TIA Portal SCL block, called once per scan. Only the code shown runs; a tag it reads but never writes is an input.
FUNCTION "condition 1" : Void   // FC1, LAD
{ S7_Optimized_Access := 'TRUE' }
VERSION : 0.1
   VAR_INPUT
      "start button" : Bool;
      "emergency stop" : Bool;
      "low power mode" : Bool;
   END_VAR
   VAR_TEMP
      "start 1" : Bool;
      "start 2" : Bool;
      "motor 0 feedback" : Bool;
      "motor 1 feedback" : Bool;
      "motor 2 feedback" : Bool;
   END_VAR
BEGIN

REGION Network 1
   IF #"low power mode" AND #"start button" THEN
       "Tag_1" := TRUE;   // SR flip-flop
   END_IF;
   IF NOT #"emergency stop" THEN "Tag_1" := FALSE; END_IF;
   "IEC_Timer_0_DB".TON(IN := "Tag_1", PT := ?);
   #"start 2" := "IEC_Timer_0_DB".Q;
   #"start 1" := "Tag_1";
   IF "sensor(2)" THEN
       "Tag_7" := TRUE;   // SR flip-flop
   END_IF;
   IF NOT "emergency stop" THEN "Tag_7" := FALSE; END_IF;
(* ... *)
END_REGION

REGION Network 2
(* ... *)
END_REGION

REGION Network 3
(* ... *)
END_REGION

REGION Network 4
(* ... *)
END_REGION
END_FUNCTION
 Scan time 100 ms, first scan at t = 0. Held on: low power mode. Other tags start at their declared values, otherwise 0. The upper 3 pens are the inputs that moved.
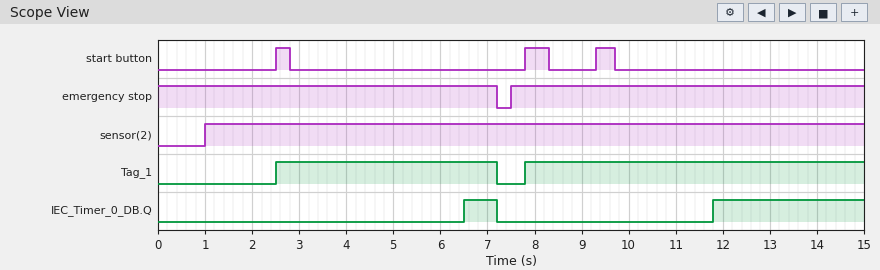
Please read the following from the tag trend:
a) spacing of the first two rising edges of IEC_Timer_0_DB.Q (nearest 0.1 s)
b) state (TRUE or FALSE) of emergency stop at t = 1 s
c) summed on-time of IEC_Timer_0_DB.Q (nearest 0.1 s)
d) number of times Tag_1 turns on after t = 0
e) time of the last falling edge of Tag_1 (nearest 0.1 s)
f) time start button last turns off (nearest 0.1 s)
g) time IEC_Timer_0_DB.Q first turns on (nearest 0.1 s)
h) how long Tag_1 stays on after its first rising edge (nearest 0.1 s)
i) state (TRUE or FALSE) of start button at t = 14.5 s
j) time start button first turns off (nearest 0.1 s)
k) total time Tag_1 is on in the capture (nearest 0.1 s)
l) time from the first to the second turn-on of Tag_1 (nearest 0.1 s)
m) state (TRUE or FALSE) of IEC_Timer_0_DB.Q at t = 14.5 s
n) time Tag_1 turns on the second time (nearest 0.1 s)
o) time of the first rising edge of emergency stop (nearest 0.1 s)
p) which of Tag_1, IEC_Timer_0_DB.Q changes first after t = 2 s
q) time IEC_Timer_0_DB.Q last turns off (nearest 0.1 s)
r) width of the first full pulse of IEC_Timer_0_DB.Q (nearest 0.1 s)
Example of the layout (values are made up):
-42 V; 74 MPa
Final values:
5.3 s; TRUE; 3.9 s; 2; 7.2 s; 9.7 s; 6.5 s; 4.7 s; FALSE; 2.8 s; 11.9 s; 5.3 s; TRUE; 7.8 s; 7.5 s; Tag_1; 7.2 s; 0.7 s
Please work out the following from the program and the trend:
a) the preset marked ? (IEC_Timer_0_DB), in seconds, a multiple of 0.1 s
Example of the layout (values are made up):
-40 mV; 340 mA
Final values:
4.0 s
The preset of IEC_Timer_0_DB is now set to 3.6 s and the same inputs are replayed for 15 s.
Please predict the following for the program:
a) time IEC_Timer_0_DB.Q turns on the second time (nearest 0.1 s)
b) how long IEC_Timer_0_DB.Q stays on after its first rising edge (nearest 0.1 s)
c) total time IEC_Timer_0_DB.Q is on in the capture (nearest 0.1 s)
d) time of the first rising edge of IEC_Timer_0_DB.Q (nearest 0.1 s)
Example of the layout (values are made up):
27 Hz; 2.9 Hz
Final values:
11.4 s; 1.1 s; 4.7 s; 6.1 s
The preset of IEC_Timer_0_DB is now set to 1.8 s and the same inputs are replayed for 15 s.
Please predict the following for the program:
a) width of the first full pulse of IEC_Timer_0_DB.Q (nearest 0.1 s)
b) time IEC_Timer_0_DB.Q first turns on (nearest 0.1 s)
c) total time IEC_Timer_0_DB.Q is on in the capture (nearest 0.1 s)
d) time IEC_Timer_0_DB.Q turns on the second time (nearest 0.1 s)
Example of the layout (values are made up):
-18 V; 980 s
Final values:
2.9 s; 4.3 s; 8.3 s; 9.6 s
